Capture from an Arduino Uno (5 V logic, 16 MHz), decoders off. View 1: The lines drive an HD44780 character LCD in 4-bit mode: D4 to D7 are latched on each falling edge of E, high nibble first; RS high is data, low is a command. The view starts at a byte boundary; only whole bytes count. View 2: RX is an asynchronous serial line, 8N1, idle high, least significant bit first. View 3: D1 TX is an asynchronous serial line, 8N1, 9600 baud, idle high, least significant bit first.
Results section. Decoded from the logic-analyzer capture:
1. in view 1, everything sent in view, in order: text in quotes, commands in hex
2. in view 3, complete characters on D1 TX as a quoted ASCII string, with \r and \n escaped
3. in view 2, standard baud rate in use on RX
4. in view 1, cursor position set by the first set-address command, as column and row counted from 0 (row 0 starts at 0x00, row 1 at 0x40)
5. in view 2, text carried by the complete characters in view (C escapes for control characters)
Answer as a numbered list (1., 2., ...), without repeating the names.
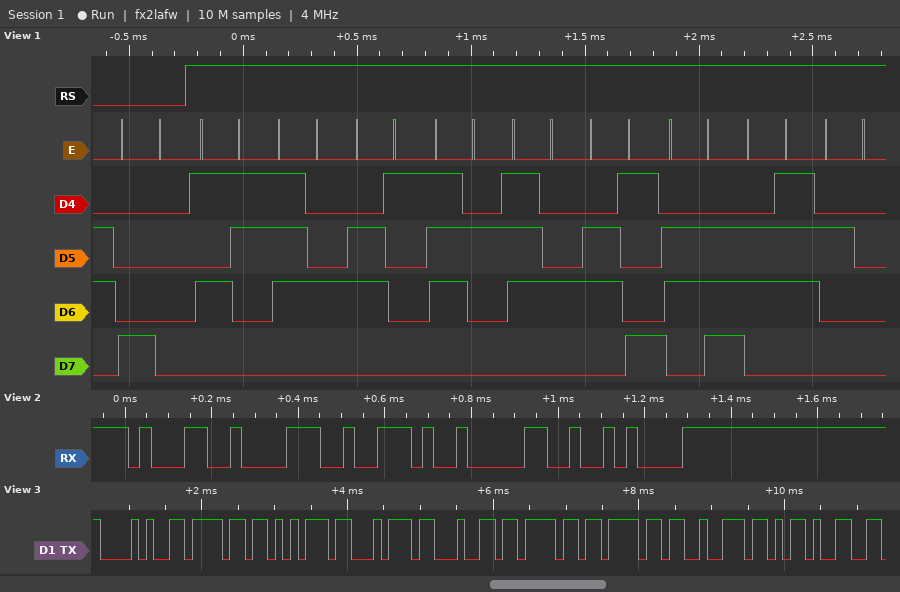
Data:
1. 0x80 "Starting "
2. "(outdoor-"
3. 38400 baud
4. column 0, row 0
5. "18.0\n"
